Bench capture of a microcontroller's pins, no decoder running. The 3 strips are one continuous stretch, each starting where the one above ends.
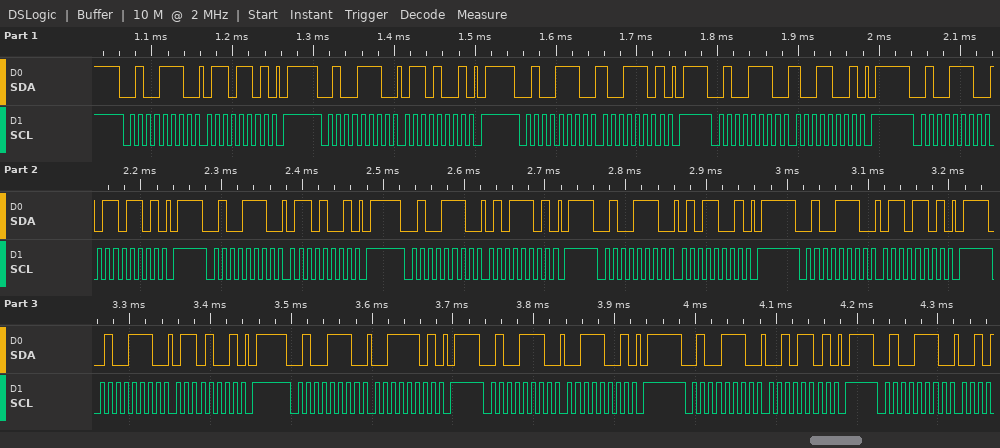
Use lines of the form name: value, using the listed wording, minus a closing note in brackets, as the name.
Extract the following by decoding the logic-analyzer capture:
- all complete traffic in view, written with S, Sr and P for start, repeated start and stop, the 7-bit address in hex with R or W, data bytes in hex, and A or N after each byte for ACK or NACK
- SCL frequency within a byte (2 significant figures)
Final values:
all complete traffic in view, written with S, Sr and P for start, repeated start and stop, the 7-bit address in hex with R or W, data bytes in hex, and A or N after each byte for ACK or NACK: S 27W A 6D A P S 27W A 69 A P S 27W A 9D A P S 27W A 99 A P S 27W A 6D A P S 27W A 69 A P S 27W A 5D A P S 27W A 59 A P S 27W A 6D A P S 27W A 69 A P S 27W A 3D A P S 27W A 39 A P S 27W A 2D A P S 27W A
SCL frequency within a byte: 100 kHz
